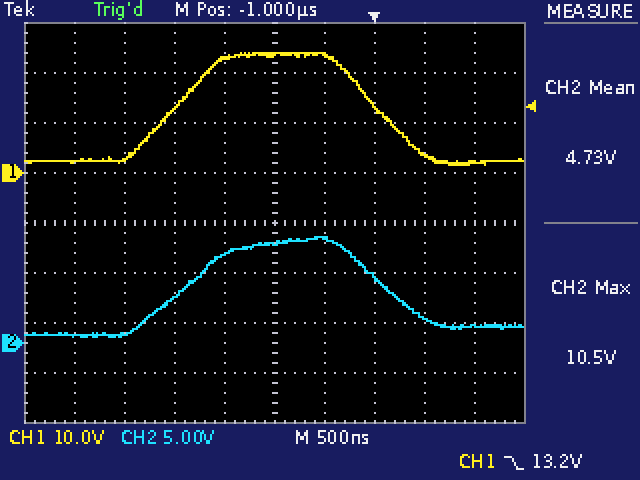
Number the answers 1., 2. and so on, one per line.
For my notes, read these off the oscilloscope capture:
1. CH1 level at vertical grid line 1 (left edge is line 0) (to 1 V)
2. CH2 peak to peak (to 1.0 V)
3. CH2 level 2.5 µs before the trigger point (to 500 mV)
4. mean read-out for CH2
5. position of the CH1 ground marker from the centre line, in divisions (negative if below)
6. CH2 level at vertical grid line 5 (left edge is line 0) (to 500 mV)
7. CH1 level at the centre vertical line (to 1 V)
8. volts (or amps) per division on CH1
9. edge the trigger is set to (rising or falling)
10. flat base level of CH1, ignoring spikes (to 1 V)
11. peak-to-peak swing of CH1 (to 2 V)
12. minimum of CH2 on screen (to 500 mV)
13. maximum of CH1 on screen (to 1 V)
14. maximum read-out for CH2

1. 2 V
2. 10.0 V
3. 1.0 V
4. 4.73 V
5. +1.0 div
6. 10.0 V
7. 24 V
8. 10 V
9. falling
10. 2 V
11. 22 V
12. 500 mV
13. 24 V
14. 10.5 V
